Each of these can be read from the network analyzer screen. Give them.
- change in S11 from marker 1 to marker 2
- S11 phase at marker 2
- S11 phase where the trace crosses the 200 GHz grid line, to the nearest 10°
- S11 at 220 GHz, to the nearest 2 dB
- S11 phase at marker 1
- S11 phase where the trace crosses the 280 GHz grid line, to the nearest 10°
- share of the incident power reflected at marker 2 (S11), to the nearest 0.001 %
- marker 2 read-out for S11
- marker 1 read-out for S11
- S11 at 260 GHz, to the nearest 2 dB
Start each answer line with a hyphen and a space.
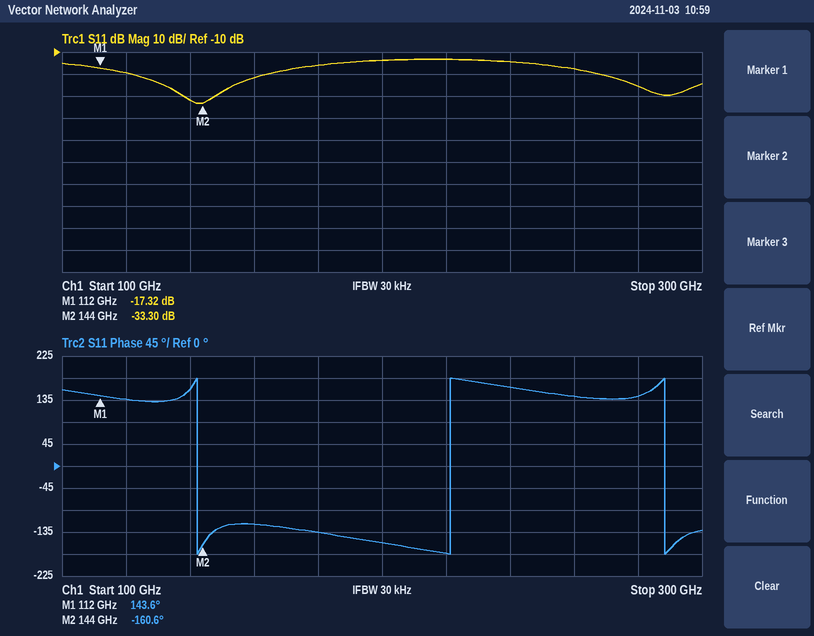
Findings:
- -15.98 dB
- -160.6°
- -160°
- -14 dB
- 143.6°
- 140°
- 0.047 %
- -33.30 dB
- -17.32 dB
- -18 dB
